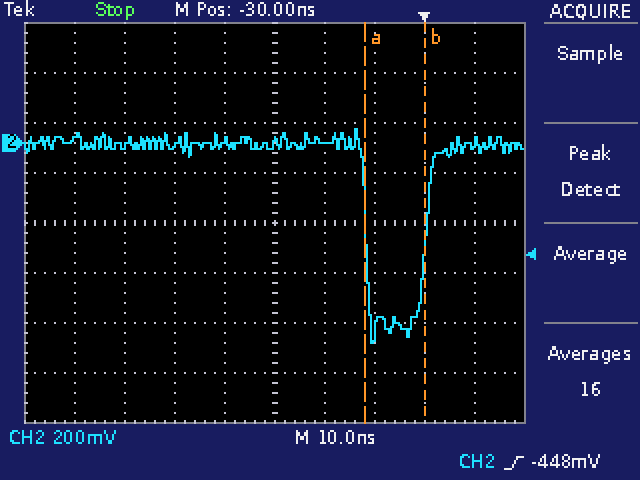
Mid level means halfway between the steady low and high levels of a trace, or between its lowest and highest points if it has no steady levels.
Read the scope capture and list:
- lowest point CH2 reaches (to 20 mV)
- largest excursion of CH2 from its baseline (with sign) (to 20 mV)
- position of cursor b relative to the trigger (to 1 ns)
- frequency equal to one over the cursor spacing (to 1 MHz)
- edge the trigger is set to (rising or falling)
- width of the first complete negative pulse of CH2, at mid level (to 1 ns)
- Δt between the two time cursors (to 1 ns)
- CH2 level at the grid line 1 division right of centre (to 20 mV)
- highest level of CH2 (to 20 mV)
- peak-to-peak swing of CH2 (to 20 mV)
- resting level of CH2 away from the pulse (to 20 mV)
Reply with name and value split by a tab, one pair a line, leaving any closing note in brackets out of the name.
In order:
lowest point CH2 reaches	-800 mV
largest excursion of CH2 from its baseline (with sign)	-800 mV
position of cursor b relative to the trigger	0 ns
frequency equal to one over the cursor spacing	83 MHz
edge the trigger is set to	rising
width of the first complete negative pulse of CH2, at mid level	12 ns
Δt between the two time cursors	12 ns
CH2 level at the grid line 1 division right of centre	0 mV
highest level of CH2	60 mV
peak-to-peak swing of CH2	860 mV
resting level of CH2 away from the pulse	0 mV
